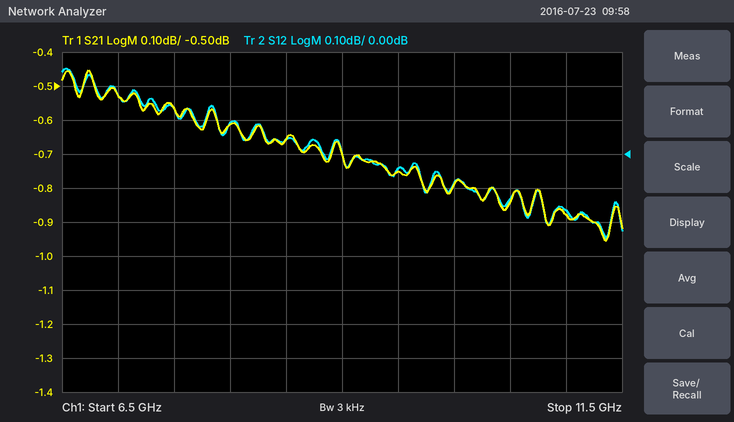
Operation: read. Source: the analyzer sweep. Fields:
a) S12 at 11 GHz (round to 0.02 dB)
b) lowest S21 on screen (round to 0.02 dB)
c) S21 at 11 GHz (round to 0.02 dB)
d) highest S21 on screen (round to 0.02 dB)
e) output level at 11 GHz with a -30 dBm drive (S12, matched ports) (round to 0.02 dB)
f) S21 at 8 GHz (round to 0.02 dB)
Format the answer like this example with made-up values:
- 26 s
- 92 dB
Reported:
- -0.16 dB
- -0.96 dB
- -0.88 dB
- -0.46 dB
- -30.16 dBm
- -0.62 dB
